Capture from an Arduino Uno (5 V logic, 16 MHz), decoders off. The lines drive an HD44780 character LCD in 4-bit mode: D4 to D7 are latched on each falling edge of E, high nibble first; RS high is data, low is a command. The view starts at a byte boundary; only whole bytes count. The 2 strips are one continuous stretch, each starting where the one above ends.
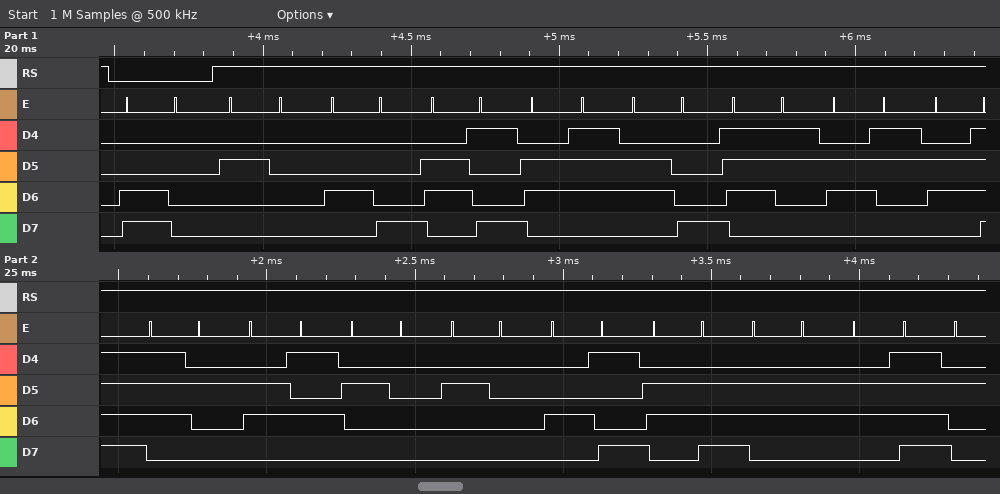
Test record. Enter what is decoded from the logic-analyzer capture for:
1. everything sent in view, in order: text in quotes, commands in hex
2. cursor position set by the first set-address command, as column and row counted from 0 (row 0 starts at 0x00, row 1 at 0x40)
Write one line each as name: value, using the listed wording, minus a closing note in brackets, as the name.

everything sent in view, in order: text in quotes, commands in hex: 0xC0 " Highscore  Info"
cursor position set by the first set-address command, as column and row counted from 0: column 0, row 1
